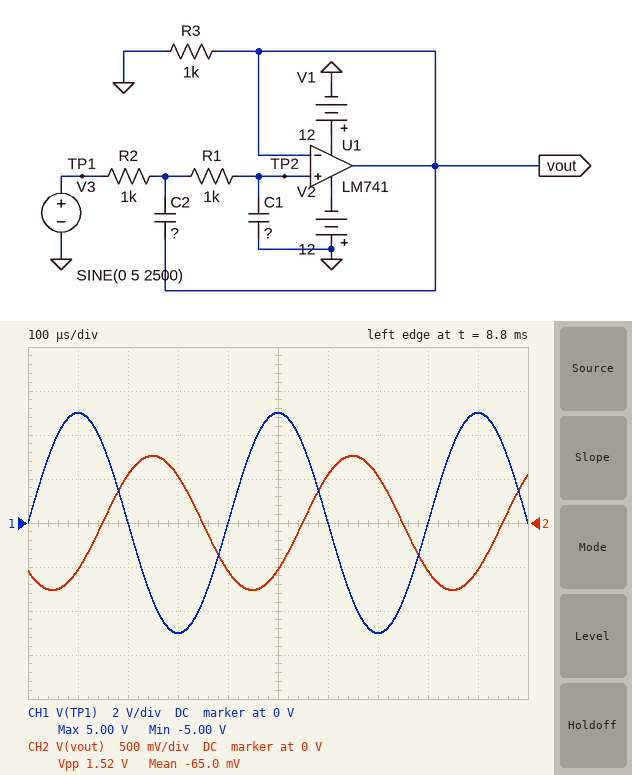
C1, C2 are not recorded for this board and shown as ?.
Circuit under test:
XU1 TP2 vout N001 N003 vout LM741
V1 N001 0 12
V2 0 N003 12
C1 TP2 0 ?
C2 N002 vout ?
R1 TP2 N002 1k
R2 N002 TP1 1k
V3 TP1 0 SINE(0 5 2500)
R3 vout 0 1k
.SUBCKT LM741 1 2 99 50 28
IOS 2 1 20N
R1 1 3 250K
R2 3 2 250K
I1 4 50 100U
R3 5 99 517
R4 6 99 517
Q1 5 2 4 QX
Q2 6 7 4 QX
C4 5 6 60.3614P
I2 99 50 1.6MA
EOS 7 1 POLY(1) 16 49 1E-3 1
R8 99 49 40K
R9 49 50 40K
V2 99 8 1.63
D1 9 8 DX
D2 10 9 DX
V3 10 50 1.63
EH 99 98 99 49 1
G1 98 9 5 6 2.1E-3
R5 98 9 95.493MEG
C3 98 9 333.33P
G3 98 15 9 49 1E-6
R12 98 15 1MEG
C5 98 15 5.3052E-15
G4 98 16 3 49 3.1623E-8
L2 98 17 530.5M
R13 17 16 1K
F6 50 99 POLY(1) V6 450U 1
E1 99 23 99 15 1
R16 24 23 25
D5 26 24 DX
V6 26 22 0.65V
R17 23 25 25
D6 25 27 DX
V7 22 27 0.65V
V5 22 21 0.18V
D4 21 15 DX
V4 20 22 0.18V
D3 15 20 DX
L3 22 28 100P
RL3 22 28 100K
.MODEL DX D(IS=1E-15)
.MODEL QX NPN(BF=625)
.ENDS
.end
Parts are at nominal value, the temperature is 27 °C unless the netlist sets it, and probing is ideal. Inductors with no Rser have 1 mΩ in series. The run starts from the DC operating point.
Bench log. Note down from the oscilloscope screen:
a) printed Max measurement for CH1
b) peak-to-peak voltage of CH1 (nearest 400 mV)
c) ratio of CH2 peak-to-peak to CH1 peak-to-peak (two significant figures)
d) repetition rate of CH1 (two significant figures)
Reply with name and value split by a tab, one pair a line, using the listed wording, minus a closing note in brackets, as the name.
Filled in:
printed Max measurement for CH1	5.00 V
peak-to-peak voltage of CH1	10.0 V
ratio of CH2 peak-to-peak to CH1 peak-to-peak	0.15
repetition rate of CH1	2.5 kHz
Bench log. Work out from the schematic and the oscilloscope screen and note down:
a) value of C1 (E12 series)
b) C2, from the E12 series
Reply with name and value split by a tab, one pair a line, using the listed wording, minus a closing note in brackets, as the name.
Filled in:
value of C1	150 nF
C2, from the E12 series	150 nF
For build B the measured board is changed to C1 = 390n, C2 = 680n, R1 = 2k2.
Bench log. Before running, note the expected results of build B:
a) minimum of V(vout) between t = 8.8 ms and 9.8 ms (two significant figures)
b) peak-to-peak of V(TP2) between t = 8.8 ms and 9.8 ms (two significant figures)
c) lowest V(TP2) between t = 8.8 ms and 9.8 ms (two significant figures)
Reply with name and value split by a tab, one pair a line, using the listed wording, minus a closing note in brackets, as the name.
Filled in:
minimum of V(vout) between t = 8.8 ms and 9.8 ms	-34 mV
peak-to-peak of V(TP2) between t = 8.8 ms and 9.8 ms	69 mV
lowest V(TP2) between t = 8.8 ms and 9.8 ms	-35 mV
